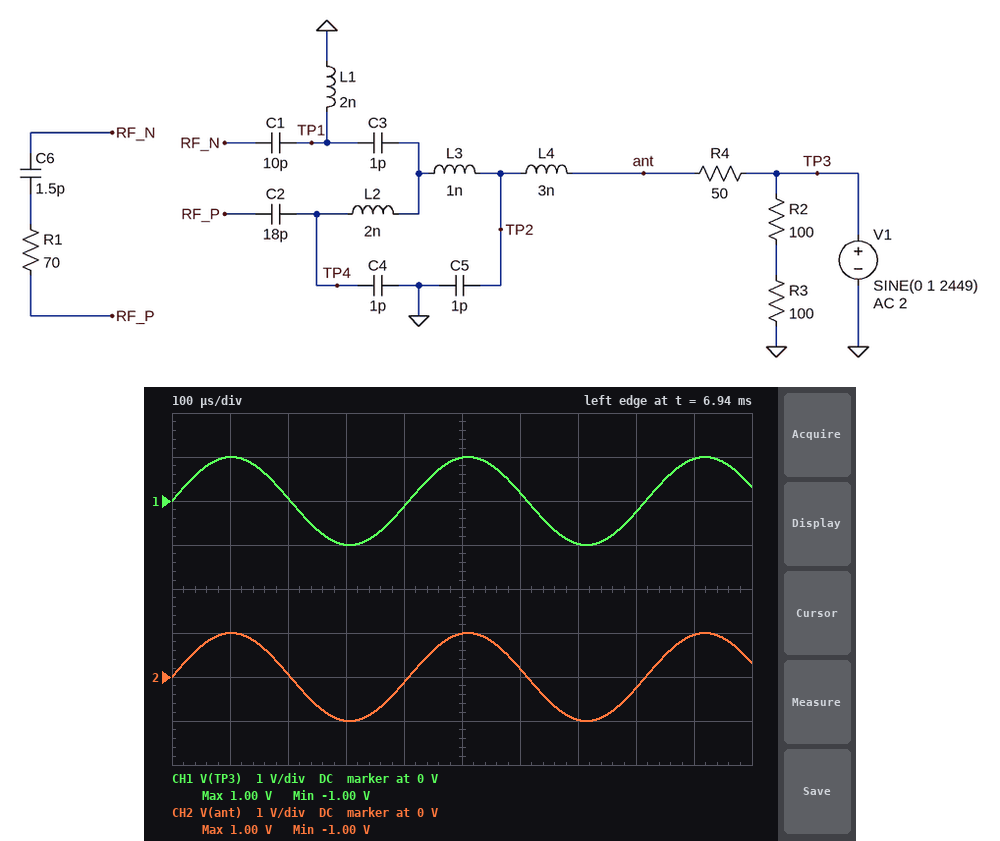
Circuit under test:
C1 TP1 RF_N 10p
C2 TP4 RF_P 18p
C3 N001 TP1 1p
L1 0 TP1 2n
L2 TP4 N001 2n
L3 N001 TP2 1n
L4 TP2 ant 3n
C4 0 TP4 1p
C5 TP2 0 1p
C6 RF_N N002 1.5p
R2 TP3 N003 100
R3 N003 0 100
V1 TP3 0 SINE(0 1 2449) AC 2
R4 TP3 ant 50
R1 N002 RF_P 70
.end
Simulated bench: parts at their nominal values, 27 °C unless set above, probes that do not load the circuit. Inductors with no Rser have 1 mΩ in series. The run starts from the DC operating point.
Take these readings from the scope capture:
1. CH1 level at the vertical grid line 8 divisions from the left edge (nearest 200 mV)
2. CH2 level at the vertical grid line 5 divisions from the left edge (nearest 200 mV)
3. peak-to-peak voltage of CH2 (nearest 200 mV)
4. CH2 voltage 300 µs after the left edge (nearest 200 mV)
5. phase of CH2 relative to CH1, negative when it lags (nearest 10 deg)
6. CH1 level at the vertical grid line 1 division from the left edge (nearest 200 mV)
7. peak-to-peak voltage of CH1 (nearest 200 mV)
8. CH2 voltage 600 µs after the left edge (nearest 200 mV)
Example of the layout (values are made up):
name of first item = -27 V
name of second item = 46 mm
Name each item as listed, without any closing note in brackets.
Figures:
CH1 level at the vertical grid line 8 divisions from the left edge = -200 mV
CH2 level at the vertical grid line 5 divisions from the left edge = 1.0 V
peak-to-peak voltage of CH2 = 2.0 V
CH2 voltage 300 µs after the left edge = -1.0 V
phase of CH2 relative to CH1, negative when it lags = 0 deg
CH1 level at the vertical grid line 1 division from the left edge = 1.0 V
peak-to-peak voltage of CH1 = 2.0 V
CH2 voltage 600 µs after the left edge = 200 mV
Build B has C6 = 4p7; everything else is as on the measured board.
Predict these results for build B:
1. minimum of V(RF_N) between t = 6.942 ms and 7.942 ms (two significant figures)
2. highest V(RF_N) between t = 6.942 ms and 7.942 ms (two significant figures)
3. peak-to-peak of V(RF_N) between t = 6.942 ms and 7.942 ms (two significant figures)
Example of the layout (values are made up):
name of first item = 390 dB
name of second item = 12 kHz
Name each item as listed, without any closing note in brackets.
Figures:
minimum of V(RF_N) between t = 6.942 ms and 7.942 ms = -270 mV
highest V(RF_N) between t = 6.942 ms and 7.942 ms = 270 mV
peak-to-peak of V(RF_N) between t = 6.942 ms and 7.942 ms = 540 mV
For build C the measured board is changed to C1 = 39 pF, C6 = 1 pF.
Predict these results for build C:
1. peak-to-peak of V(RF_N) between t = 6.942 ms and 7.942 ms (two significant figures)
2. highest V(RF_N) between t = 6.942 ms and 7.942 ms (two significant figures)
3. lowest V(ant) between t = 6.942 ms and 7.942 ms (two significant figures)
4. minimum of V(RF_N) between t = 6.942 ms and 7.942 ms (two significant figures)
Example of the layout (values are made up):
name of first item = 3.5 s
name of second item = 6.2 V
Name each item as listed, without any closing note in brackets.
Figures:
peak-to-peak of V(RF_N) between t = 6.942 ms and 7.942 ms = 47 mV
highest V(RF_N) between t = 6.942 ms and 7.942 ms = 24 mV
lowest V(ant) between t = 6.942 ms and 7.942 ms = -1.0 V
minimum of V(RF_N) between t = 6.942 ms and 7.942 ms = -24 mV
